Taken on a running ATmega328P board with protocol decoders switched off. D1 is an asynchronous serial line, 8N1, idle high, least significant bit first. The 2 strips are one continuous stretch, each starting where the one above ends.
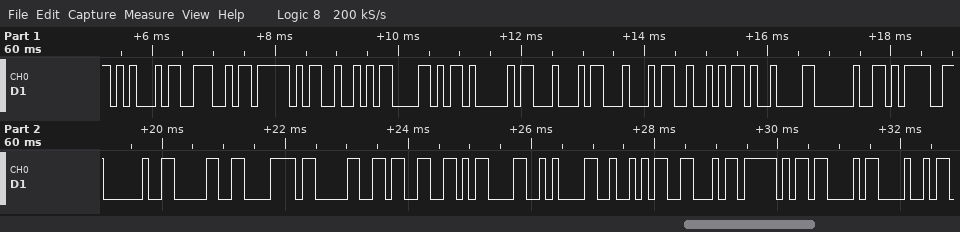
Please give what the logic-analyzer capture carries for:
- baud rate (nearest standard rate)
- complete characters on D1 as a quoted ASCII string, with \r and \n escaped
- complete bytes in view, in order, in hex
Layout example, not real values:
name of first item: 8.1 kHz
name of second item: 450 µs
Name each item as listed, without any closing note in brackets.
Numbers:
baud rate: 9600 baud
complete characters on D1 as a quoted ASCII string, with \r and \n escaped: "EN_RXADDR\t = 0x03\r\nRF_CH"
complete bytes in view, in order, in hex: 0x45 0x4E 0x5F 0x52 0x58 0x41 0x44 0x44 0x52 0x09 0x20 0x3D 0x20 0x30 0x78 0x30 0x33 0x0D 0x0A 0x52 0x46 0x5F 0x43 0x48
